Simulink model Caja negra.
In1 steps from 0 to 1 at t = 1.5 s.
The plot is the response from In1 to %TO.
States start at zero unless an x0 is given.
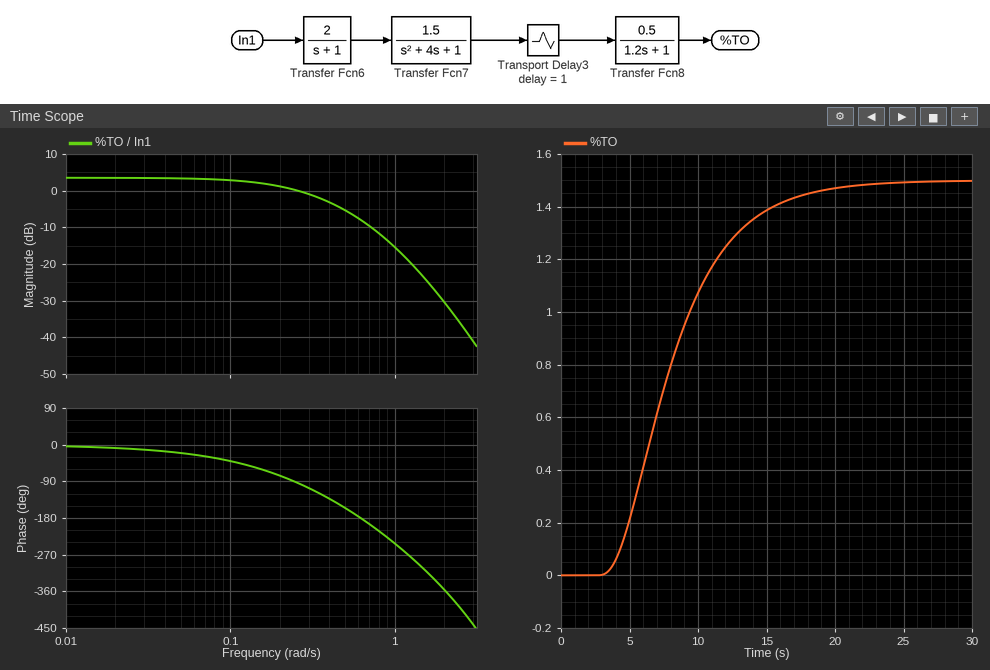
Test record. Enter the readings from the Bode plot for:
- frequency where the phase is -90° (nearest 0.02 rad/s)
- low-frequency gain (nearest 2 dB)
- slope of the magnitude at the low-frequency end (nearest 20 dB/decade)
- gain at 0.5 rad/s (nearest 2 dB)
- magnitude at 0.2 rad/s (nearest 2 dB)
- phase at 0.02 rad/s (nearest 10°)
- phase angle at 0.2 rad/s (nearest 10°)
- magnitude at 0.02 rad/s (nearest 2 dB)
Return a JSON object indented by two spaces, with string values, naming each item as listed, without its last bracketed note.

{
  "frequency where the phase is -90°": "0.24 rad/s",
  "low-frequency gain": "4 dB",
  "slope of the magnitude at the low-frequency end": "0 dB/decade",
  "gain at 0.5 rad/s": "-6 dB",
  "magnitude at 0.2 rad/s": "2 dB",
  "phase at 0.02 rad/s": "-10°",
  "phase angle at 0.2 rad/s": "-80°",
  "magnitude at 0.02 rad/s": "4 dB"
}
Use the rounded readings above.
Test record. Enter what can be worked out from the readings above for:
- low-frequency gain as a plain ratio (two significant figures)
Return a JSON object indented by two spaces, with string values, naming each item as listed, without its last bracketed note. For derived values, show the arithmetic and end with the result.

{
  "low-frequency gain as a plain ratio": "10^(4 / 20) = 1.6"
}
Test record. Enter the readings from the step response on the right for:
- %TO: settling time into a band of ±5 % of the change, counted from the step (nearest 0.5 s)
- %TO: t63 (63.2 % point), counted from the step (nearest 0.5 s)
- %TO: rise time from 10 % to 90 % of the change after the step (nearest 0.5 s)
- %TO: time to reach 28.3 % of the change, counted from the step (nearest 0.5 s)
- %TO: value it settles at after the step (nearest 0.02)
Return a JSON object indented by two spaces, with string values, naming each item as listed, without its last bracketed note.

{
  "%TO: settling time into a band of ±5 % of the change, counted from the step": "15.0 s",
  "%TO: t63 (63.2 % point), counted from the step": "7.5 s",
  "%TO: rise time from 10 % to 90 % of the change after the step": "9.5 s",
  "%TO: time to reach 28.3 % of the change, counted from the step": "4.5 s",
  "%TO: value it settles at after the step": "1.50"
}
